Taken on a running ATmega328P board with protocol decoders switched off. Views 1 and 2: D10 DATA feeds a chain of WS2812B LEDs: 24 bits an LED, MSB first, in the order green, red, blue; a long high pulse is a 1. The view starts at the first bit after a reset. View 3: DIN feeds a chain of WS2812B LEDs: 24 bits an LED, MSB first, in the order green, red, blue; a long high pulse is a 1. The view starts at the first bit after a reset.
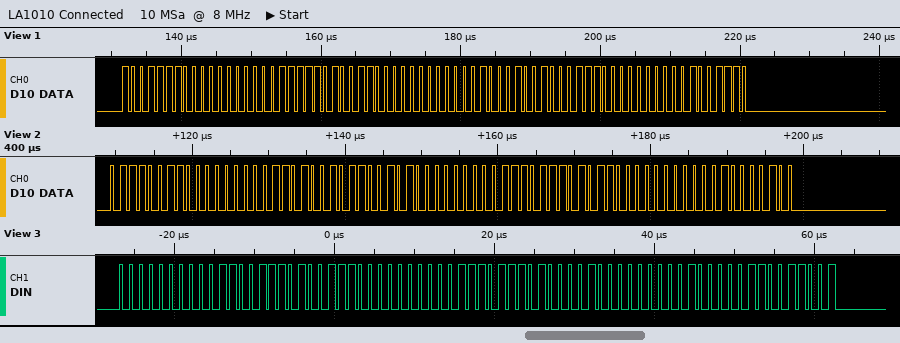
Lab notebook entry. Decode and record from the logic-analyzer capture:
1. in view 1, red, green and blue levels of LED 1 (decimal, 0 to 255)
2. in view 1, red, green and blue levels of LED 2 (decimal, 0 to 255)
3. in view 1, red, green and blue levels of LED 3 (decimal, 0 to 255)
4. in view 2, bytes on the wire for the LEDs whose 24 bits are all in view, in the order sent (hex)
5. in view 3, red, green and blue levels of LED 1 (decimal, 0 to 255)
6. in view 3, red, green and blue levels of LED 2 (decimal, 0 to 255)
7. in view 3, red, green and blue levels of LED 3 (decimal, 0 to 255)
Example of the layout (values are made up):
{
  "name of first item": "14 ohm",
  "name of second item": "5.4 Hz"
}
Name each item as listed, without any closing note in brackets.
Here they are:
{
  "in view 1, red, green and blue levels of LED 1": "0, 158, 62",
  "in view 1, red, green and blue levels of LED 2": "0, 152, 68",
  "in view 1, red, green and blue levels of LED 3": "0, 142, 78",
  "in view 2, bytes on the wire for the LEDs whose 24 bits are all in view, in the order sent": "73 00 69 65 00 77 58 00 84",
  "in view 3, red, green and blue levels of LED 1": "51, 0, 167",
  "in view 3, red, green and blue levels of LED 2": "59, 0, 161",
  "in view 3, red, green and blue levels of LED 3": "65, 0, 153"
}
